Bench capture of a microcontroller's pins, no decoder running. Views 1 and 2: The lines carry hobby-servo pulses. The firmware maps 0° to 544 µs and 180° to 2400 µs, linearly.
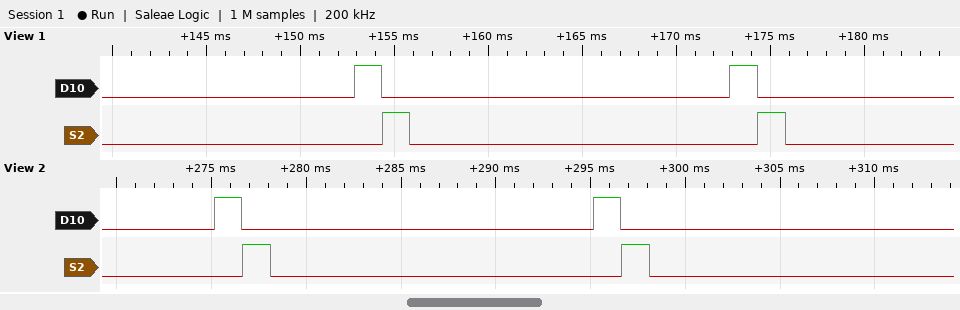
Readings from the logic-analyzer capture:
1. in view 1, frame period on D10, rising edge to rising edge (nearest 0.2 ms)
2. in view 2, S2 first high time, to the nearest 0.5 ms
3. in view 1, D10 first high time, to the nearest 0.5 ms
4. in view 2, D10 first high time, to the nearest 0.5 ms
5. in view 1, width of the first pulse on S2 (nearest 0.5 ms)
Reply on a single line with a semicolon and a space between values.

20.0 ms; 1.5 ms; 1.5 ms; 1.5 ms; 1.5 ms
